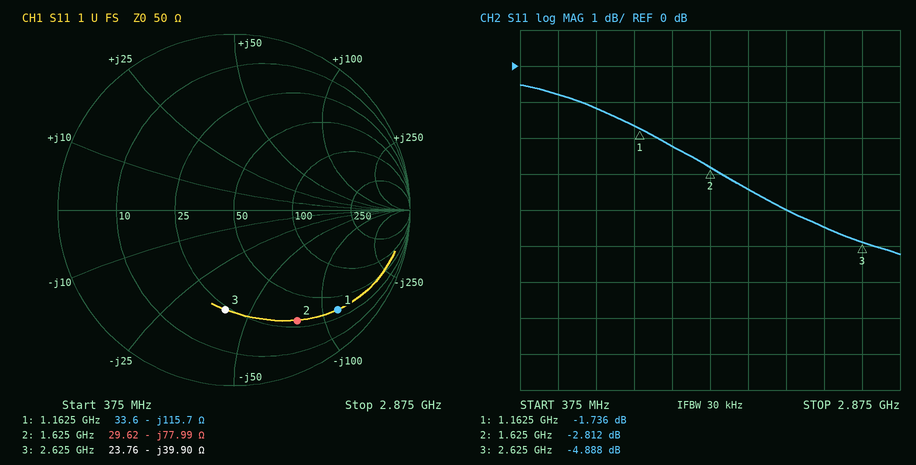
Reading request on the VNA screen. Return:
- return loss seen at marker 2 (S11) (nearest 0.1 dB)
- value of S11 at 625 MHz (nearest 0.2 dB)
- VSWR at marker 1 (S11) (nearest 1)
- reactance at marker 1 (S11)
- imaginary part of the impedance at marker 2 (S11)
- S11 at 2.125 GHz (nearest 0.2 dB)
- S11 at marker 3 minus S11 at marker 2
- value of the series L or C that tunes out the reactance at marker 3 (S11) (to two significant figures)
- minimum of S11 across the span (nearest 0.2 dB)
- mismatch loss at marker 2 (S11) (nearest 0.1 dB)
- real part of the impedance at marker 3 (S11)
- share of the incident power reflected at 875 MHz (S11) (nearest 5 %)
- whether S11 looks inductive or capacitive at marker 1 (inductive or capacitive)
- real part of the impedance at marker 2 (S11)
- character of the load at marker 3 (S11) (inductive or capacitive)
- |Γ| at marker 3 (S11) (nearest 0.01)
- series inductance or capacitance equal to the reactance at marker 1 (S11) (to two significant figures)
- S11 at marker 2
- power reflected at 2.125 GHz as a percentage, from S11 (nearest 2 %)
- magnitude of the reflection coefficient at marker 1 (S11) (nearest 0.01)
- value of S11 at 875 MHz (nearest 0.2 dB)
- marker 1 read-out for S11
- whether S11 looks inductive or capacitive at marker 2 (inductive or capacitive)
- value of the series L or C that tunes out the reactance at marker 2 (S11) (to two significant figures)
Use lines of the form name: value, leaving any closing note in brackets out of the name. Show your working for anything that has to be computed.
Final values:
return loss seen at marker 2 (S11): 2.8 dB
value of S11 at 625 MHz: -0.8 dB
VSWR at marker 1 (S11): 10
reactance at marker 1: -115.7 Ω
imaginary part of the impedance at marker 2: -77.99 Ω
S11 at 2.125 GHz: -4.0 dB
S11 at marker 3 minus S11 at marker 2: -4.888 − (-2.812) = -2.076 dB
value of the series L or C that tunes out the reactance at marker 3 (S11): L = 39.9 Ω/(2π × 2.625 GHz) ≈ 2.4 nH
minimum of S11 across the span: -5.2 dB
mismatch loss at marker 2 (S11): −10 log10(1 − 10^(-2.812/10)) ≈ 3.2 dB
real part of the impedance at marker 3: 23.76 Ω
share of the incident power reflected at 875 MHz (S11): 10^(-1.2/10) ≈ 75.9 %, so 75 % to the nearest 5 %
whether S11 looks inductive or capacitive at marker 1: capacitive
real part of the impedance at marker 2: 29.62 Ω
character of the load at marker 3 (S11): capacitive
|Γ| at marker 3 (S11): 0.57
series inductance or capacitance equal to the reactance at marker 1 (S11): C = 1/(2π × 1.1625 GHz × 115.7 Ω) ≈ 1.2 pF
S11 at marker 2: -2.812 dB
power reflected at 2.125 GHz as a percentage, from S11: 10^(-4/10) ≈ 40 %
magnitude of the reflection coefficient at marker 1 (S11): 10^(-1.736/20) ≈ 0.82
value of S11 at 875 MHz: -1.2 dB
marker 1 read-out for S11: -1.736 dB
whether S11 looks inductive or capacitive at marker 2: capacitive
value of the series L or C that tunes out the reactance at marker 2 (S11): L = 77.99 Ω/(2π × 1.625 GHz) ≈ 7.6 nH
